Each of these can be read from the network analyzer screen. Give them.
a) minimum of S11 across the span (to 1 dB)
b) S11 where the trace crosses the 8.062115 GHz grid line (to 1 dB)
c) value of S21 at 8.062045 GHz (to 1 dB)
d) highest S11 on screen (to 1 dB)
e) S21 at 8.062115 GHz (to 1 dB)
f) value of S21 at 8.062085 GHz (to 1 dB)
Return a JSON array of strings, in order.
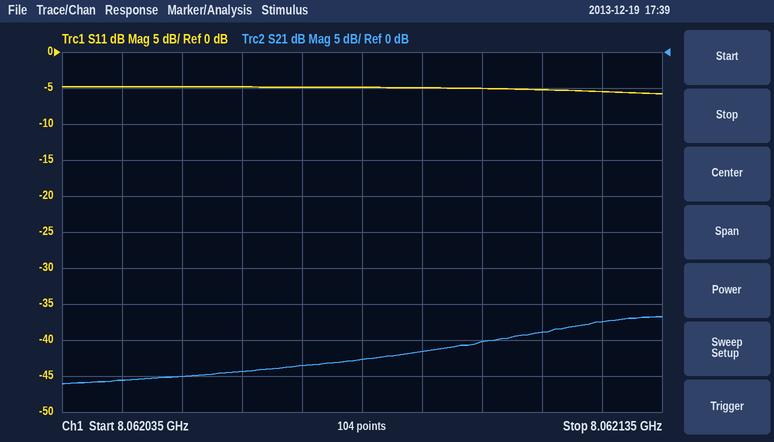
["-6 dB", "-5 dB", "-46 dB", "-5 dB", "-39 dB", "-43 dB"]
